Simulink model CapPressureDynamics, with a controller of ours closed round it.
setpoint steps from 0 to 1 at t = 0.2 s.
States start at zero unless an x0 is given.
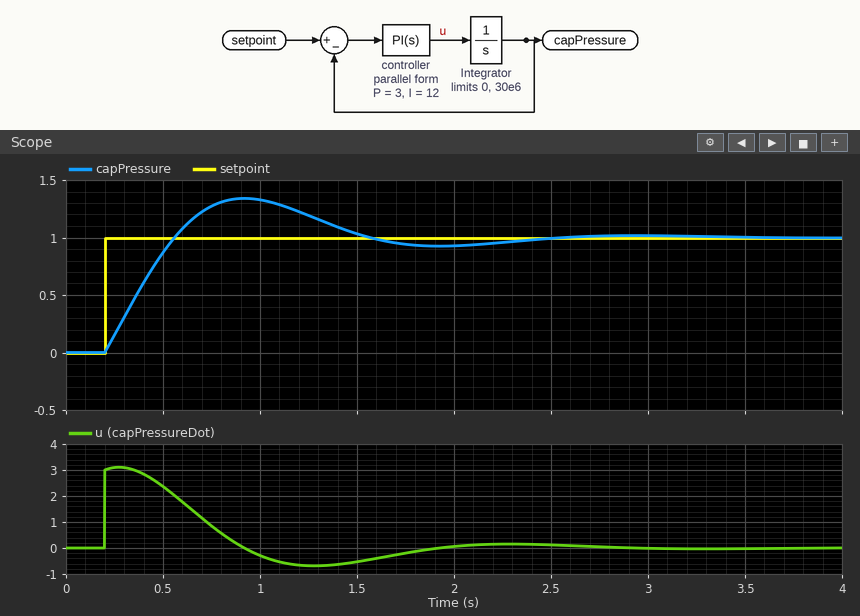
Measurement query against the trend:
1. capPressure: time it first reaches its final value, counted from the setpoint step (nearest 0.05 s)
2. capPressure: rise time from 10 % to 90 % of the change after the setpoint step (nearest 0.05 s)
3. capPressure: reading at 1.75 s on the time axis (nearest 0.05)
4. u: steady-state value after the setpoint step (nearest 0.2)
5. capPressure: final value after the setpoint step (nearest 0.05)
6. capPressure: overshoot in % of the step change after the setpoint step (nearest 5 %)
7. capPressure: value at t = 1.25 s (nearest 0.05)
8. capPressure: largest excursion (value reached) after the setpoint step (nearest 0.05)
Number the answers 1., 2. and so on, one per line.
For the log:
1. 0.35 s
2. 0.30 s
3. 0.95
4. 0.0
5. 1.00
6. 35 %
7. 1.20
8. 1.35
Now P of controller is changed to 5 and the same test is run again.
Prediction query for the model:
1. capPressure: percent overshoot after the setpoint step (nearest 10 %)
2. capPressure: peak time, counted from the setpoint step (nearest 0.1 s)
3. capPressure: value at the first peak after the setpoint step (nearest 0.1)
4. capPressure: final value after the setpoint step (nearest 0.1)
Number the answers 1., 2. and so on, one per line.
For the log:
1. 20 %
2. 0.6 s
3. 1.2
4. 1.0
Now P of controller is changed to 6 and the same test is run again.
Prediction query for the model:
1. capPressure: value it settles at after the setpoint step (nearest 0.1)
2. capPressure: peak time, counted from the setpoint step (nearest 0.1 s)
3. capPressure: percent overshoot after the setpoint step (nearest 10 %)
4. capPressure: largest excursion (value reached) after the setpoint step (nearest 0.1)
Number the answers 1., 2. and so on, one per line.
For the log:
1. 1.0
2. 0.6 s
3. 20 %
4. 1.2
